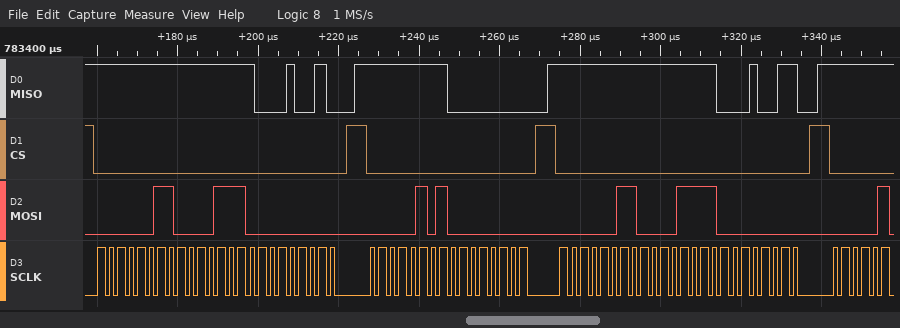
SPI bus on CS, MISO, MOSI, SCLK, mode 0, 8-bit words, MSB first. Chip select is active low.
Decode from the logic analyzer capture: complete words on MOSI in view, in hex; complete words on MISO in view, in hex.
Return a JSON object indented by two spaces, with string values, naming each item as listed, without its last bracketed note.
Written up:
{
  "complete words on MOSI in view, in hex": "03, 0E, 00, 05, 00, 03, 0F, 00",
  "complete words on MISO in view, in hex": "FF, FF, 12, FF, 00, FF, FF, 13"
}
